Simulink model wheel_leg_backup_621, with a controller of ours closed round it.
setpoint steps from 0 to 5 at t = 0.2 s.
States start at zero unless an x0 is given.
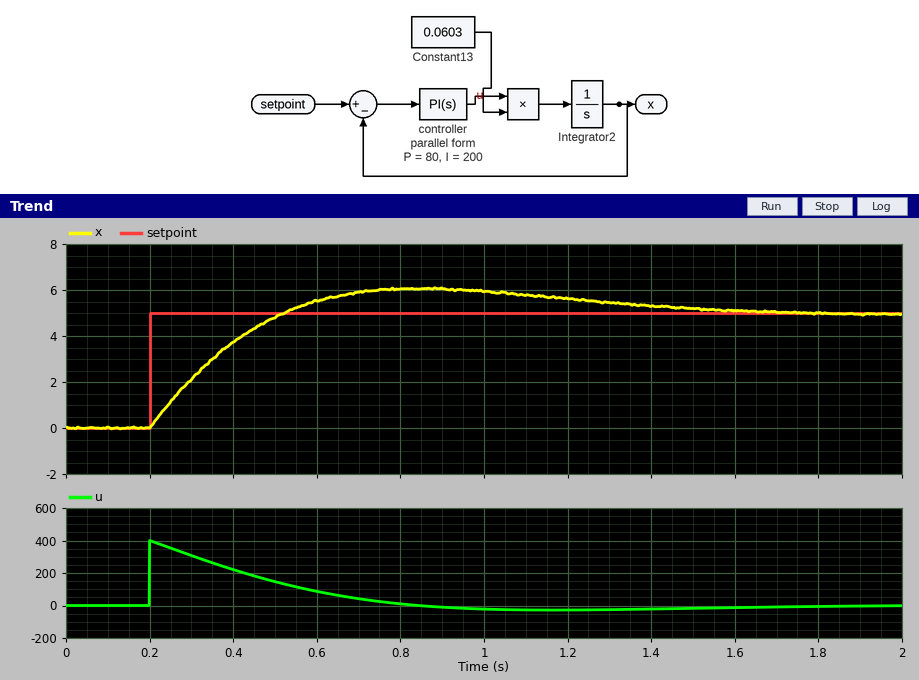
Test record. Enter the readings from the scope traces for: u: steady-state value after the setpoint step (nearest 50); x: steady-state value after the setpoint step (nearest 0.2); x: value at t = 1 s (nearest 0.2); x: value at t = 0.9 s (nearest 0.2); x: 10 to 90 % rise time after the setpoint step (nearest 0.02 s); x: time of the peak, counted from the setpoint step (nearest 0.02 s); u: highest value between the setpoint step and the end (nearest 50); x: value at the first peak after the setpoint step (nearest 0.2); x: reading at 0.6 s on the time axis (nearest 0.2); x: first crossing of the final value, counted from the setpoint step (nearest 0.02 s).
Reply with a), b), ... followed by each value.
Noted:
a) 0
b) 5.0
c) 6.0
d) 6.0
e) 0.24 s
f) 0.64 s
g) 400
h) 6.0
i) 5.6
j) 0.32 s
